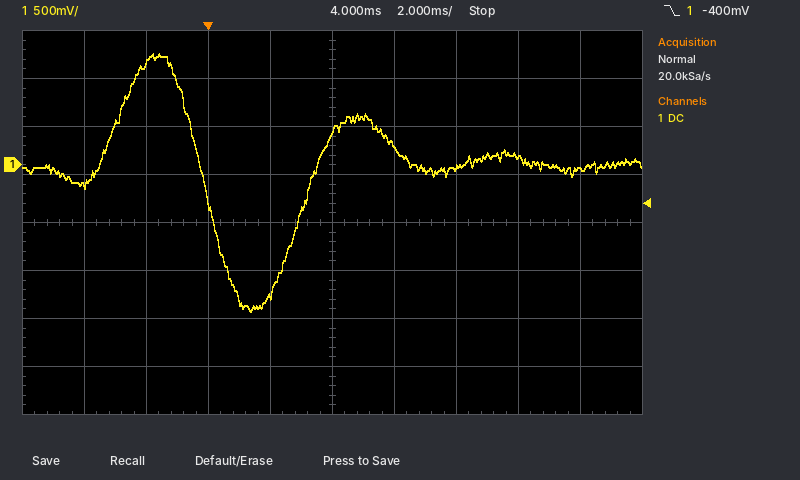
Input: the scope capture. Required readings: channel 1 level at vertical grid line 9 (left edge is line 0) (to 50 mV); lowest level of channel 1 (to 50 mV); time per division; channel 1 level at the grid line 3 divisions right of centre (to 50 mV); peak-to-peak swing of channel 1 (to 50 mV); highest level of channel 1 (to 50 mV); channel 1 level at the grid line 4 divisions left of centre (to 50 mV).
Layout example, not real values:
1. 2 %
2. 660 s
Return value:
1. -50 mV
2. -1.55 V
3. 2 ms
4. 100 mV
5. 2.70 V
6. 1.15 V
7. -200 mV
